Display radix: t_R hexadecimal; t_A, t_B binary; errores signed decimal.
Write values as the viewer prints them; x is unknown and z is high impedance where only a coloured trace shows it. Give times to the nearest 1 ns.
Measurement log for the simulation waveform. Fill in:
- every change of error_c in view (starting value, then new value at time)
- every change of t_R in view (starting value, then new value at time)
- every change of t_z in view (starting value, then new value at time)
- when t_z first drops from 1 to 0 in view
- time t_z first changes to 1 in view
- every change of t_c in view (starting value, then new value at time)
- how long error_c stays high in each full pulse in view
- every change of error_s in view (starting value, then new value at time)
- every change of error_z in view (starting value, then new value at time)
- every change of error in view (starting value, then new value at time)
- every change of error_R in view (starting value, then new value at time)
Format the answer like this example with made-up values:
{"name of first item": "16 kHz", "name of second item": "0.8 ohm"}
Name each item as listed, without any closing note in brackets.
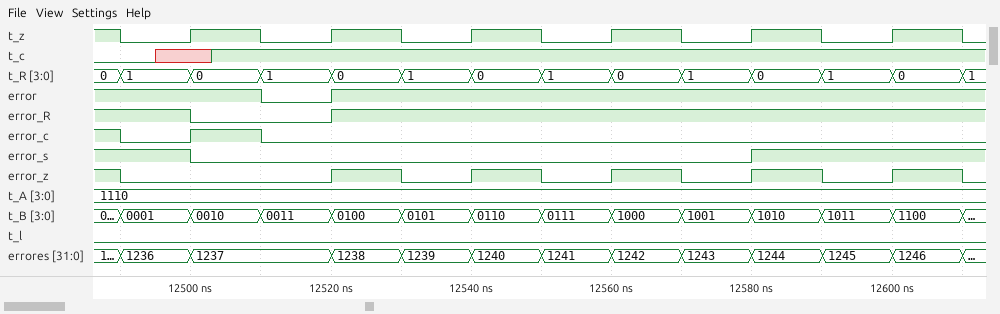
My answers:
{"every change of error_c in view": "1, 0 at 12490 ns, 1 at 12500 ns, 0 at 12510 ns", "every change of t_R in view": "0, 1 at 12490 ns, 0 at 12500 ns, 1 at 12510 ns, 0 at 12520 ns, 1 at 12530 ns, 0 at 12540 ns, 1 at 12550 ns, 0 at 12560 ns, 1 at 12570 ns, 0 at 12580 ns, 1 at 12590 ns, 0 at 12600 ns, 1 at 12610 ns", "every change of t_z in view": "1, 0 at 12490 ns, 1 at 12500 ns, 0 at 12510 ns, 1 at 12520 ns, 0 at 12530 ns, 1 at 12540 ns, 0 at 12550 ns, 1 at 12560 ns, 0 at 12570 ns, 1 at 12580 ns, 0 at 12590 ns, 1 at 12600 ns, 0 at 12610 ns", "when t_z first drops from 1 to 0 in view": "12490 ns", "time t_z first changes to 1 in view": "12500 ns", "every change of t_c in view": "0, x at 12495 ns, 1 at 12503 ns", "how long error_c stays high in each full pulse in view": "10 ns", "every change of error_s in view": "1, 0 at 12500 ns, 1 at 12580 ns", "every change of error_z in view": "1, 0 at 12490 ns, 1 at 12520 ns, 0 at 12530 ns, 1 at 12540 ns, 0 at 12550 ns, 1 at 12560 ns, 0 at 12570 ns, 1 at 12580 ns, 0 at 12590 ns, 1 at 12600 ns, 0 at 12610 ns", "every change of error in view": "1, 0 at 12510 ns, 1 at 12520 ns", "every change of error_R in view": "1, 0 at 12500 ns, 1 at 12520 ns"}
